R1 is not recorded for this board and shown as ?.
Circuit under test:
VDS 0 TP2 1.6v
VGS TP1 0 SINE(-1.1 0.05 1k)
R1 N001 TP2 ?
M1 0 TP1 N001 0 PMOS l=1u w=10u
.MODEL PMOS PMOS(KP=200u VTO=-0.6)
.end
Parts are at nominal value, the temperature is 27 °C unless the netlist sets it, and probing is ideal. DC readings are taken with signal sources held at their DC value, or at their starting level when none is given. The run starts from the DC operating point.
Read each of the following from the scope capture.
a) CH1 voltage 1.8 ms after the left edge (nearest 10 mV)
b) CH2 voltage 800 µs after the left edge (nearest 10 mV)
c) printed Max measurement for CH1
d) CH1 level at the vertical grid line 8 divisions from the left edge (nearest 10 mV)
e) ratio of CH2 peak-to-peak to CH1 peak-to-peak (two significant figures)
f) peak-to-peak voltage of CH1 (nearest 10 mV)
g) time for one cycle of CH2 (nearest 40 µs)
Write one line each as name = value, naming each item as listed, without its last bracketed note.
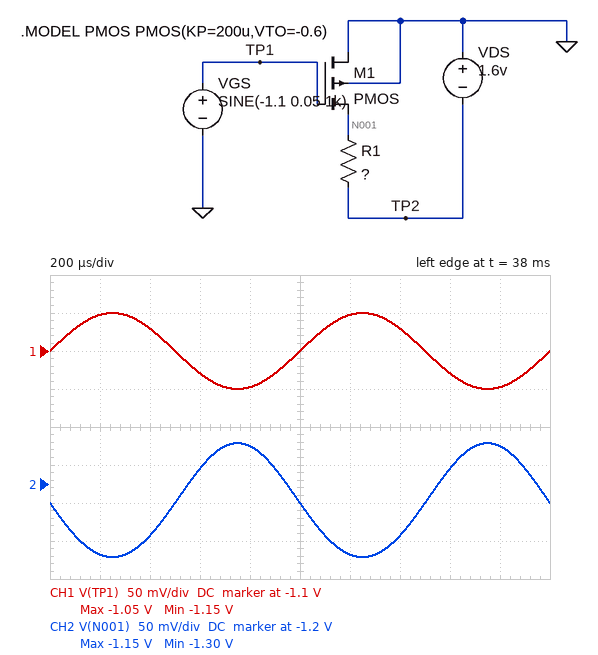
CH1 voltage 1.8 ms after the left edge = -1.15 V
CH2 voltage 800 µs after the left edge = -1.15 V
printed Max measurement for CH1 = -1.05 V
CH1 level at the vertical grid line 8 divisions from the left edge = -1.13 V
ratio of CH2 peak-to-peak to CH1 peak-to-peak = 1.5
peak-to-peak voltage of CH1 = 100 mV
time for one cycle of CH2 = 1.00 ms
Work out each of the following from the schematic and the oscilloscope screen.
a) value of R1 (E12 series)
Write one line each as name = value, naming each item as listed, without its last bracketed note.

value of R1 = 1.5 kΩ
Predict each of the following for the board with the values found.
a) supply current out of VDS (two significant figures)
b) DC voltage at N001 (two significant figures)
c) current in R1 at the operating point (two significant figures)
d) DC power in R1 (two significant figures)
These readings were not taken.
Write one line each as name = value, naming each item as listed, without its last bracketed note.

supply current out of VDS = 250 µA
DC voltage at N001 = -1.2 V
current in R1 at the operating point = 250 µA
DC power in R1 = 94 µW
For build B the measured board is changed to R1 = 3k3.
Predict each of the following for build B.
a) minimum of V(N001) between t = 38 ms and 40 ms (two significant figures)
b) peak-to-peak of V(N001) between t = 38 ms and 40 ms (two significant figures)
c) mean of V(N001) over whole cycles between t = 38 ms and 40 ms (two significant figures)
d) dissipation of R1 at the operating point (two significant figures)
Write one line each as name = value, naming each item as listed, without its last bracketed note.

minimum of V(N001) between t = 38 ms and 40 ms = -930 mV
peak-to-peak of V(N001) between t = 38 ms and 40 ms = 330 mV
mean of V(N001) over whole cycles between t = 38 ms and 40 ms = -770 mV
dissipation of R1 at the operating point = 210 µW
